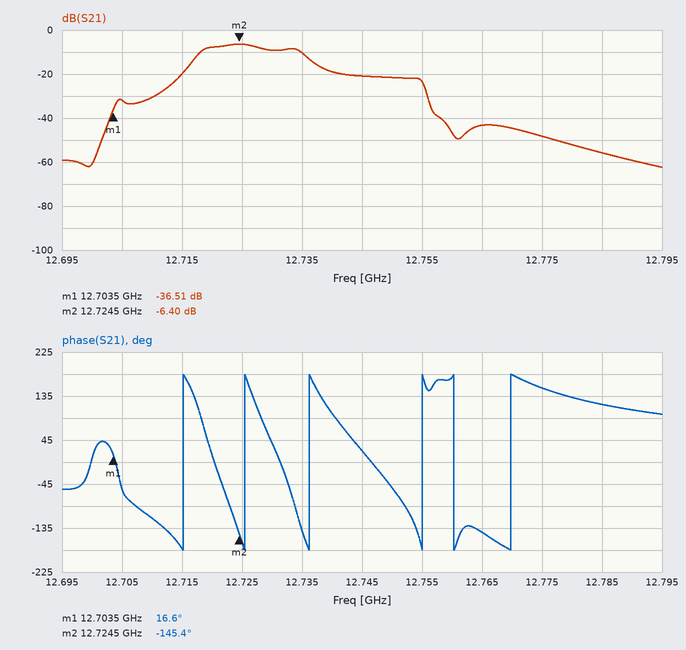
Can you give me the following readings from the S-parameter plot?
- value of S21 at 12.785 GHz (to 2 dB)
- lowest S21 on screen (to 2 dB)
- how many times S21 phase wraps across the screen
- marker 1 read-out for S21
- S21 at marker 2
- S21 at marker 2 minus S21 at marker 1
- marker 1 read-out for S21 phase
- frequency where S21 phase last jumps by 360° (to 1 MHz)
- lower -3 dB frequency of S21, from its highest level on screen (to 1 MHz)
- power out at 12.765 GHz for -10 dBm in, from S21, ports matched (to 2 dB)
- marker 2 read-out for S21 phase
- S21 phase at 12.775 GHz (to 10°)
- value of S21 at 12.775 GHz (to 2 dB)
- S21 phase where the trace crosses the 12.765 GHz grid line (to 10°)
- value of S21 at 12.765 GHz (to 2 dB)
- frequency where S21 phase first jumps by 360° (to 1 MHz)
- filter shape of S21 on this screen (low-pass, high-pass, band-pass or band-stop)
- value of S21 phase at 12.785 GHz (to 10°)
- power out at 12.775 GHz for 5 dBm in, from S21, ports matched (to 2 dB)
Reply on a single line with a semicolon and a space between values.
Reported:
-56 dB; -62 dB; 6; -36.51 dB; -6.40 dB; 30.11 dB; 16.6°; 12.770 GHz; 12.718 GHz; -54 dBm; -145.4°; 150°; -48 dB; -140°; -44 dB; 12.715 GHz; band-pass; 120°; -44 dBm
